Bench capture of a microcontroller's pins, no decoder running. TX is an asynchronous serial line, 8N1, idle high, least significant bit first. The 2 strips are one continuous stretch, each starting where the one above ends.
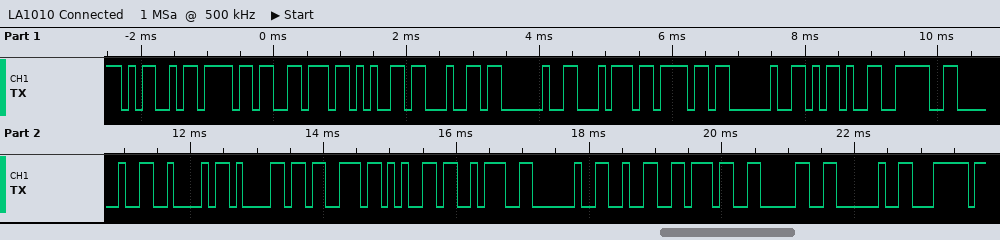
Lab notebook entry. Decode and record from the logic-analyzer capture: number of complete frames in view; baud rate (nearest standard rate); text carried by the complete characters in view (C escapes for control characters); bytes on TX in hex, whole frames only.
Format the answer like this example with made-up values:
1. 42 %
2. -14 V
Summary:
1. 23
2. 9600 baud
3. "Moved to -> Base: 270 |"
4. 0x4D 0x6F 0x76 0x65 0x64 0x20 0x74 0x6F 0x20 0x2D 0x3E 0x20 0x42 0x61 0x73 0x65 0x3A 0x20 0x32 0x37 0x30 0x20 0x7C
